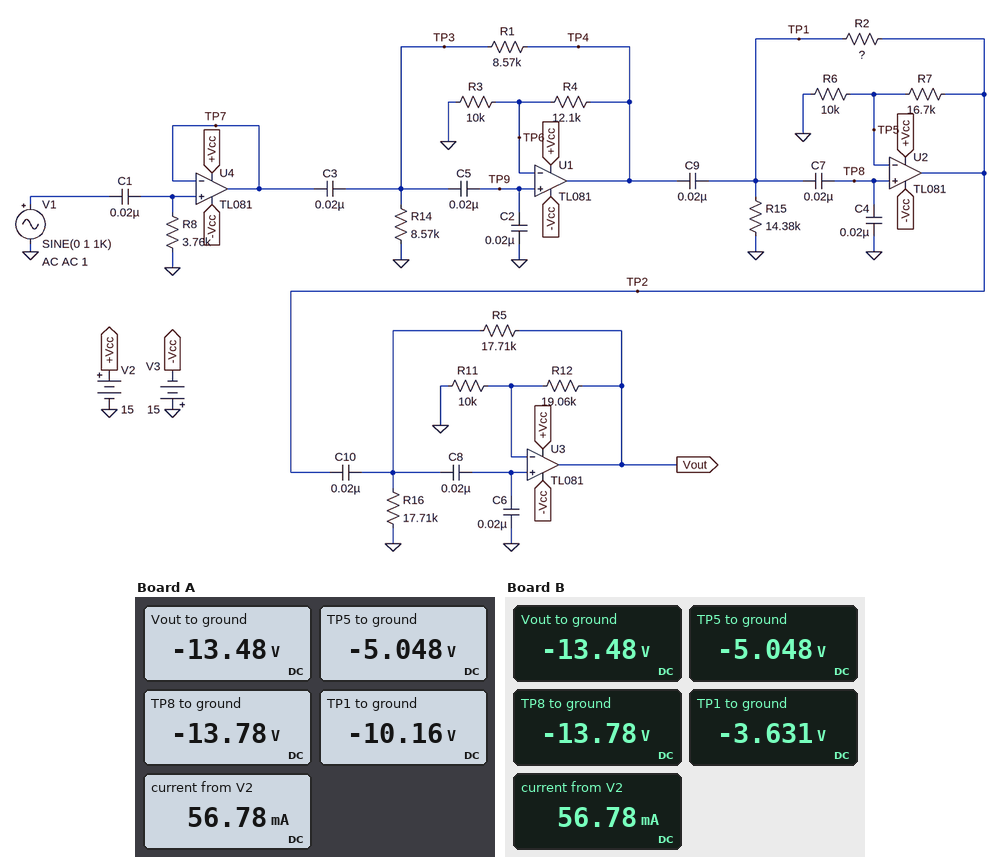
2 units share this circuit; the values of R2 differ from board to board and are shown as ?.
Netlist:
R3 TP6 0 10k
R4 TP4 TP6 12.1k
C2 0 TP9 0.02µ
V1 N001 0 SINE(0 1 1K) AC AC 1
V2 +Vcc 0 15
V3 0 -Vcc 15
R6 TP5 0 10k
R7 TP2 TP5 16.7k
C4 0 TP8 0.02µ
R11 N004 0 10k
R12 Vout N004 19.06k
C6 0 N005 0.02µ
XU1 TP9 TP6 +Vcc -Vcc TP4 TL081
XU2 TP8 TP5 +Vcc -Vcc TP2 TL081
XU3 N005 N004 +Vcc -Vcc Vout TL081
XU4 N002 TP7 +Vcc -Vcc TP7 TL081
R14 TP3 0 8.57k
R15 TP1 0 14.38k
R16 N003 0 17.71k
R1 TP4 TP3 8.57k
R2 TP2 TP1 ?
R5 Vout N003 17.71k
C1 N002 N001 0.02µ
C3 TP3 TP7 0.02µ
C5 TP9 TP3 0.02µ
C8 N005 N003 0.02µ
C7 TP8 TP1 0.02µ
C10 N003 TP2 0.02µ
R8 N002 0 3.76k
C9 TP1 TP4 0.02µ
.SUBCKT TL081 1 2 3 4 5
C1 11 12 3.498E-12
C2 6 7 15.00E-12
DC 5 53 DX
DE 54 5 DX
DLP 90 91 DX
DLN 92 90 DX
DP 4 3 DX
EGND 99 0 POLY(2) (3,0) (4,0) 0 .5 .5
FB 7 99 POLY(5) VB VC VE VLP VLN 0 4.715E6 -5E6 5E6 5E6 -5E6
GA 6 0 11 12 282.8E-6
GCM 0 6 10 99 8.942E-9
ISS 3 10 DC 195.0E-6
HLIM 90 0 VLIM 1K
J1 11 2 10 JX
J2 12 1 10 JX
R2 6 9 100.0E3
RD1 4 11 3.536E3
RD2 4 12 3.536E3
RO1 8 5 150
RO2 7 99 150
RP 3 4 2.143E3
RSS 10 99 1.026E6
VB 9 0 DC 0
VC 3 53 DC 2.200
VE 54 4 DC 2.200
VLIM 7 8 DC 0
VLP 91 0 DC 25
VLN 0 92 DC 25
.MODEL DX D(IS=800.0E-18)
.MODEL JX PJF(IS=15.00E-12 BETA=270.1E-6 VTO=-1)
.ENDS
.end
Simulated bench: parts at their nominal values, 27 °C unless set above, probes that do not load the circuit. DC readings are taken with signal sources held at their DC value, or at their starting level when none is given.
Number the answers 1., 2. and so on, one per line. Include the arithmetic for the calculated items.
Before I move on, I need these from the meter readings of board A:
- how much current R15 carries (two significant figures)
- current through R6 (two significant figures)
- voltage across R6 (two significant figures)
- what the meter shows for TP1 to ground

1. (0 V - (-10.16 V)) / 14.38 kΩ = 710 µA
2. (0 V - (-5.048 V)) / 10 kΩ = 500 µA
3. 0 V - (-5.048 V) = 5.0 V
4. -10.16 V
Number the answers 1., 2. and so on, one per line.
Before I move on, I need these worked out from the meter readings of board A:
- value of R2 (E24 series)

1. 4.7 kΩ
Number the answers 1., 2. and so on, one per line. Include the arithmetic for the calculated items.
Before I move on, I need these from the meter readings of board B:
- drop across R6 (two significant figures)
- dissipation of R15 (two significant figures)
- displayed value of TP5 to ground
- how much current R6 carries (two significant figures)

1. 0 V - (-5.048 V) = 5.0 V
2. (0 V - (-3.631 V))^2 / 14.38 kΩ = 920 µW
3. -5.048 V
4. (0 V - (-5.048 V)) / 10 kΩ = 500 µA
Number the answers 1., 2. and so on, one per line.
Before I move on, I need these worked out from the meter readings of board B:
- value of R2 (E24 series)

1. 39 kΩ
